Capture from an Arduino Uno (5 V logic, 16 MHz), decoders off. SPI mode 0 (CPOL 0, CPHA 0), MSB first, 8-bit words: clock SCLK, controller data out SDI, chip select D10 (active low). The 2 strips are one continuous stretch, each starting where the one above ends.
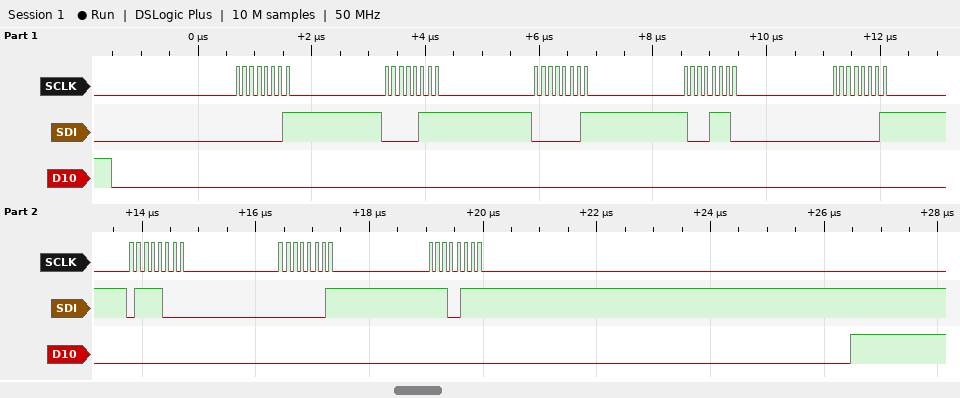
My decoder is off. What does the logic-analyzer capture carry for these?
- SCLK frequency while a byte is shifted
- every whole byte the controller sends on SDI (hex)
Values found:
8 MHz
01 07 01 8E 01 78 01 E7
